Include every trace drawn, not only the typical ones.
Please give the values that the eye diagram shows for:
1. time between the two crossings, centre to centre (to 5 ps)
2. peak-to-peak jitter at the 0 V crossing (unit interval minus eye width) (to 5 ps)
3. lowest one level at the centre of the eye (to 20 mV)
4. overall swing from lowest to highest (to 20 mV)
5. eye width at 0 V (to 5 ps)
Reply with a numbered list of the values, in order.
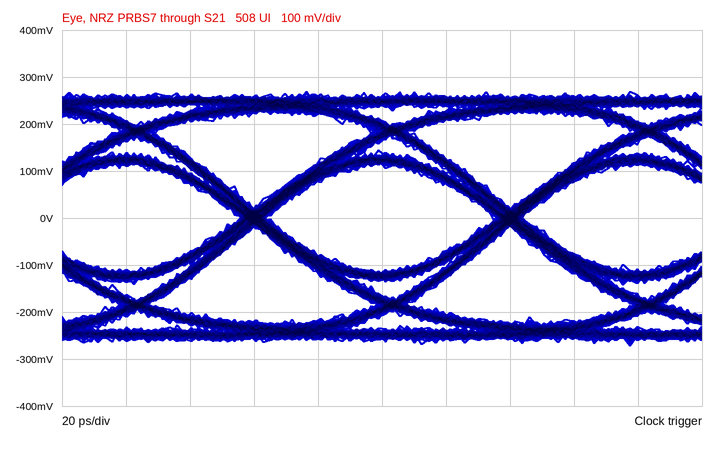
1. 80 ps
2. 10 ps
3. 120 mV
4. 540 mV
5. 70 ps
